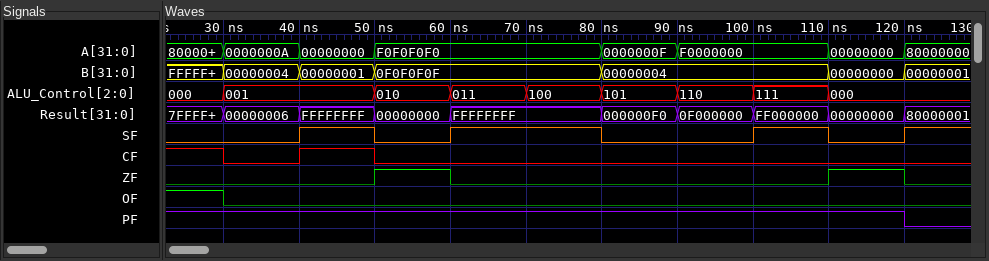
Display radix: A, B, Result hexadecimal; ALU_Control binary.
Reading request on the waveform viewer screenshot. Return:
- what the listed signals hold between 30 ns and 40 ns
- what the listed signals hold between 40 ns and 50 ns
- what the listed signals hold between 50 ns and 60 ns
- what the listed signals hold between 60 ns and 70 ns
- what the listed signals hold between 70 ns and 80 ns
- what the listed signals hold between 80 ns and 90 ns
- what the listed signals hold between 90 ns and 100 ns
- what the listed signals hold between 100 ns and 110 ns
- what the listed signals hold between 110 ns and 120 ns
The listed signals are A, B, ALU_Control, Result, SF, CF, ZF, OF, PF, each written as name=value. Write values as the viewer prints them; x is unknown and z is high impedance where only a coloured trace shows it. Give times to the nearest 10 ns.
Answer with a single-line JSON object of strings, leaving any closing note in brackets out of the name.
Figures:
{"what the listed signals hold between 30 ns and 40 ns": "A=0000000A, B=00000004, ALU_Control=001, Result=00000006, SF=0, CF=0, ZF=0, OF=0, PF=1", "what the listed signals hold between 40 ns and 50 ns": "A=00000000, B=00000001, ALU_Control=001, Result=FFFFFFFF, SF=1, CF=1, ZF=0, OF=0, PF=1", "what the listed signals hold between 50 ns and 60 ns": "A=F0F0F0F0, B=0F0F0F0F, ALU_Control=010, Result=00000000, SF=0, CF=0, ZF=1, OF=0, PF=1", "what the listed signals hold between 60 ns and 70 ns": "A=F0F0F0F0, B=0F0F0F0F, ALU_Control=011, Result=FFFFFFFF, SF=1, CF=0, ZF=0, OF=0, PF=1", "what the listed signals hold between 70 ns and 80 ns": "A=F0F0F0F0, B=0F0F0F0F, ALU_Control=100, Result=FFFFFFFF, SF=1, CF=0, ZF=0, OF=0, PF=1", "what the listed signals hold between 80 ns and 90 ns": "A=0000000F, B=00000004, ALU_Control=101, Result=000000F0, SF=0, CF=0, ZF=0, OF=0, PF=1", "what the listed signals hold between 90 ns and 100 ns": "A=F0000000, B=00000004, ALU_Control=110, Result=0F000000, SF=0, CF=0, ZF=0, OF=0, PF=1", "what the listed signals hold between 100 ns and 110 ns": "A=F0000000, B=00000004, ALU_Control=111, Result=FF000000, SF=1, CF=0, ZF=0, OF=0, PF=1", "what the listed signals hold between 110 ns and 120 ns": "A=00000000, B=00000000, ALU_Control=000, Result=00000000, SF=0, CF=0, ZF=1, OF=0, PF=1"}
